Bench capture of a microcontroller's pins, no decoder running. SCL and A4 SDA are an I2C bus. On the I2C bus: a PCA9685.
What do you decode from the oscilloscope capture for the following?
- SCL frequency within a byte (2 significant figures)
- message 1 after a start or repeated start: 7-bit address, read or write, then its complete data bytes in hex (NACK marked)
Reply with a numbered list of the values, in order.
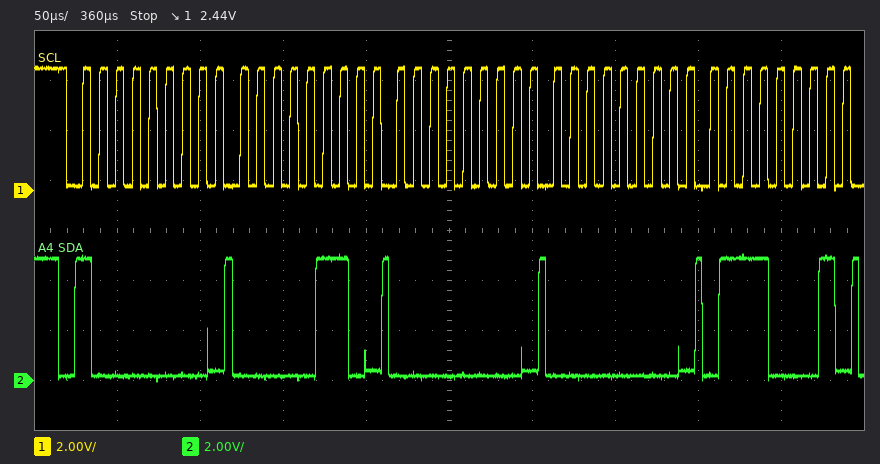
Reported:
1. 100 kHz
2. 0x40 write: 06 00 00 71
